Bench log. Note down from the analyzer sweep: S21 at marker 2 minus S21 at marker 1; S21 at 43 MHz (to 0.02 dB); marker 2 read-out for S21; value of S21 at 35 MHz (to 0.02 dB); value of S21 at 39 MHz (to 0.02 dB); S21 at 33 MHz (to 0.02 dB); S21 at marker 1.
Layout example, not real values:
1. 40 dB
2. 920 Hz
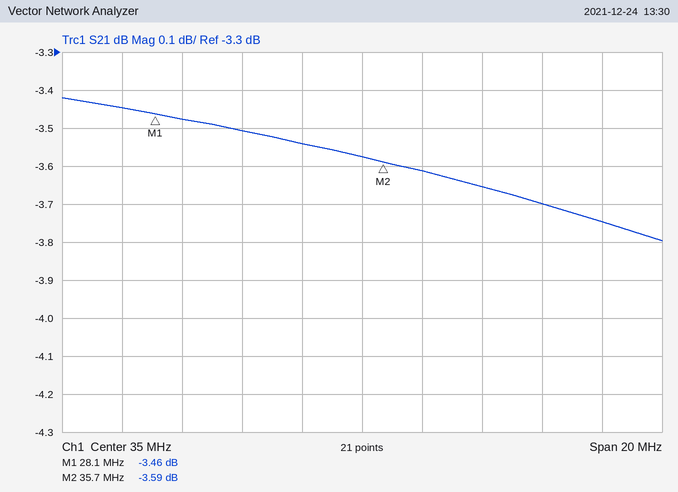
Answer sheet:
1. -0.13 dB
2. -3.74 dB
3. -3.59 dB
4. -3.58 dB
5. -3.66 dB
6. -3.54 dB
7. -3.46 dB
